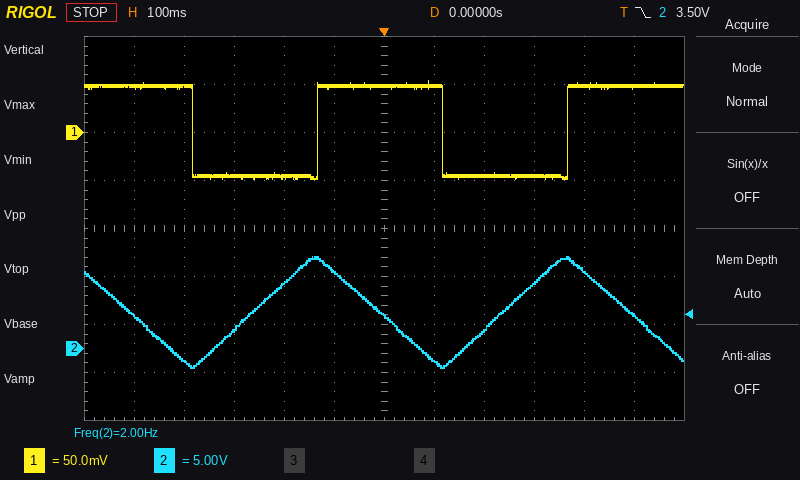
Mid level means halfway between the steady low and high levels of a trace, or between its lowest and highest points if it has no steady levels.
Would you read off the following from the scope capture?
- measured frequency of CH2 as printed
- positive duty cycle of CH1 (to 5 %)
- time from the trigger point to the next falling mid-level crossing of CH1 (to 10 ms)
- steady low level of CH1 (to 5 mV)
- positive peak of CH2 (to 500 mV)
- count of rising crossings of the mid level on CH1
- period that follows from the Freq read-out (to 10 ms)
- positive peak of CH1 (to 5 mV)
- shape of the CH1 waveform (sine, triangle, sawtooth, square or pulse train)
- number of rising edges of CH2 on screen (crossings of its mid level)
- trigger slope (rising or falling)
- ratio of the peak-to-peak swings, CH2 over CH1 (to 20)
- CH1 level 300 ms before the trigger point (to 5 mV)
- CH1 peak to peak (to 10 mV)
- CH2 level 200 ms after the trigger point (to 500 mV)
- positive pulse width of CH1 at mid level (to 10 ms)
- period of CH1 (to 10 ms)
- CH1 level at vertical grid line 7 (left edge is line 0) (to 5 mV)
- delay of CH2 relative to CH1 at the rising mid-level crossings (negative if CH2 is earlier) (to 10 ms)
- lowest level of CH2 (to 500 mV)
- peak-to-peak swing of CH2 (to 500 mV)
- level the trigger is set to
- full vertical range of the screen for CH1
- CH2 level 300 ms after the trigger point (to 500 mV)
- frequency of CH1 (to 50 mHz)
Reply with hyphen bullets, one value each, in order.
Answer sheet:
- 2.00 Hz
- 50 %
- 120 ms
- -45 mV
- 9.5 V
- 2
- 500 ms
- 55 mV
- square
- 2
- falling
- 120
- -45 mV
- 100 mV
- 2.0 V
- 250 ms
- 500 ms
- 50 mV
- -130 ms
- -2.0 V
- 11.5 V
- 3.50 V
- 400 mV
- 7.0 V
- 2.00 Hz
